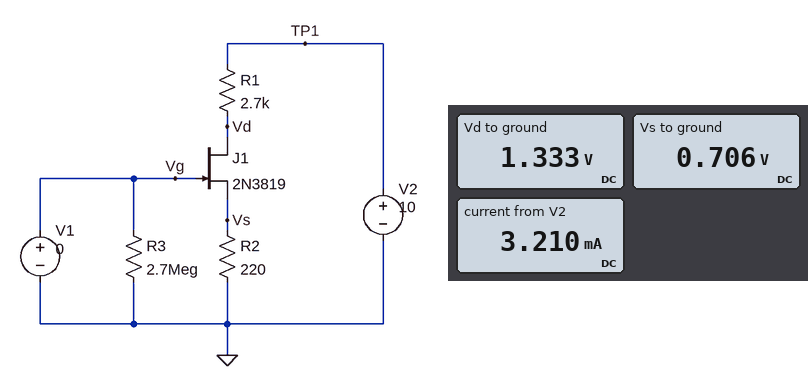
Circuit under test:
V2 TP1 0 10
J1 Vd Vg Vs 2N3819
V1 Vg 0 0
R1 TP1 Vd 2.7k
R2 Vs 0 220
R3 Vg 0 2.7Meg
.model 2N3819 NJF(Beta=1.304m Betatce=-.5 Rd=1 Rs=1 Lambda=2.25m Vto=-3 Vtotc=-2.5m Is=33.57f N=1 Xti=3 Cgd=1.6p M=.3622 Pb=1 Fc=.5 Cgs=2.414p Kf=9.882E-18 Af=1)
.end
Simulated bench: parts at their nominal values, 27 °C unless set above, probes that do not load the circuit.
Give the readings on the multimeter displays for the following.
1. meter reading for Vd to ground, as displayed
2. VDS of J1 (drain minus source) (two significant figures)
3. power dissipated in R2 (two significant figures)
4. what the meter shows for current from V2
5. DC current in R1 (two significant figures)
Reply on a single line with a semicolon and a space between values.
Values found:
1.333 V; 630 mV; 2.3 mW; 3.210 mA; 3.2 mA
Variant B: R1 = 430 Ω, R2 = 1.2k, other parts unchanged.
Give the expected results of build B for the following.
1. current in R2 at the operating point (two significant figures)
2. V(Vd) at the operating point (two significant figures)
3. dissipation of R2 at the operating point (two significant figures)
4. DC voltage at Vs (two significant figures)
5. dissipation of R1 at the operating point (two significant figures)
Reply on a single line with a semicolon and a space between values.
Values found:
1.6 mA; 9.3 V; 3.0 mW; 1.9 V; 1.1 mW
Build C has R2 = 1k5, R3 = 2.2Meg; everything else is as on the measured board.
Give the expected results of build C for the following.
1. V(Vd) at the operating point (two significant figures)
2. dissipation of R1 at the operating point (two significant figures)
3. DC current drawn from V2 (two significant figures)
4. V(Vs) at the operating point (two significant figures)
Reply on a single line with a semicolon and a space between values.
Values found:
6.4 V; 4.8 mW; 1.3 mA; 2.0 V
